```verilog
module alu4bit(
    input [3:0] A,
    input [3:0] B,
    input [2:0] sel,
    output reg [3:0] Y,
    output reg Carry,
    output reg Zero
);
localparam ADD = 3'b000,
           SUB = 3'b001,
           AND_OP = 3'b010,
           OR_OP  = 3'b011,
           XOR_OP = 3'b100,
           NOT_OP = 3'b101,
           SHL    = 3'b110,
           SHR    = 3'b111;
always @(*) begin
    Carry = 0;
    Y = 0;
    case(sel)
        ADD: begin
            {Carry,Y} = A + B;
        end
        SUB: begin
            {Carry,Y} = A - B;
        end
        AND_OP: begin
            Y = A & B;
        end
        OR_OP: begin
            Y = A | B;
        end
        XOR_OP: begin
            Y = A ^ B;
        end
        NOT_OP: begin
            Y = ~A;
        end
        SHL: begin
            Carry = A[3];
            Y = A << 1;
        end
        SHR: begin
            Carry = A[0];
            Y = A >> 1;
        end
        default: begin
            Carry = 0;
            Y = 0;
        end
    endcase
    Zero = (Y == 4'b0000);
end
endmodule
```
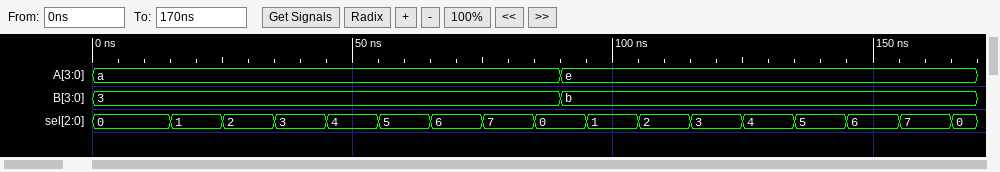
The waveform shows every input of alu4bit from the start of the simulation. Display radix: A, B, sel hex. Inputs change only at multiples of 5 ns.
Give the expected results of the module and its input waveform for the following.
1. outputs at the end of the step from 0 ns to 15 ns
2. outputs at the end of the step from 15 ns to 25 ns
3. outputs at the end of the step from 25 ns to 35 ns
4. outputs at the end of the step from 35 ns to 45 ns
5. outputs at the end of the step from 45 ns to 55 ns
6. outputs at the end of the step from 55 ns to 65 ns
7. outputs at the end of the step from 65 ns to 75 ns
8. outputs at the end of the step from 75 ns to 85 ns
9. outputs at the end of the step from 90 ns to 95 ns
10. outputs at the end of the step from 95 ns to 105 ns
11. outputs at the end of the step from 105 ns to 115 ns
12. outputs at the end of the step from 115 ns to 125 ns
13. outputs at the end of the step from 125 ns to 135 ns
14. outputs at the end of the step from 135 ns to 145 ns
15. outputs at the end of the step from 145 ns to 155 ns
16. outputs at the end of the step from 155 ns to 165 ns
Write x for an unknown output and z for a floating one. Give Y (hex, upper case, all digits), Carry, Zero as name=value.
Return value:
Y=D, Carry=0, Zero=0
Y=7, Carry=0, Zero=0
Y=2, Carry=0, Zero=0
Y=B, Carry=0, Zero=0
Y=9, Carry=0, Zero=0
Y=5, Carry=0, Zero=0
Y=4, Carry=1, Zero=0
Y=5, Carry=0, Zero=0
Y=9, Carry=1, Zero=0
Y=3, Carry=0, Zero=0
Y=A, Carry=0, Zero=0
Y=F, Carry=0, Zero=0
Y=5, Carry=0, Zero=0
Y=1, Carry=0, Zero=0
Y=C, Carry=1, Zero=0
Y=7, Carry=0, Zero=0
